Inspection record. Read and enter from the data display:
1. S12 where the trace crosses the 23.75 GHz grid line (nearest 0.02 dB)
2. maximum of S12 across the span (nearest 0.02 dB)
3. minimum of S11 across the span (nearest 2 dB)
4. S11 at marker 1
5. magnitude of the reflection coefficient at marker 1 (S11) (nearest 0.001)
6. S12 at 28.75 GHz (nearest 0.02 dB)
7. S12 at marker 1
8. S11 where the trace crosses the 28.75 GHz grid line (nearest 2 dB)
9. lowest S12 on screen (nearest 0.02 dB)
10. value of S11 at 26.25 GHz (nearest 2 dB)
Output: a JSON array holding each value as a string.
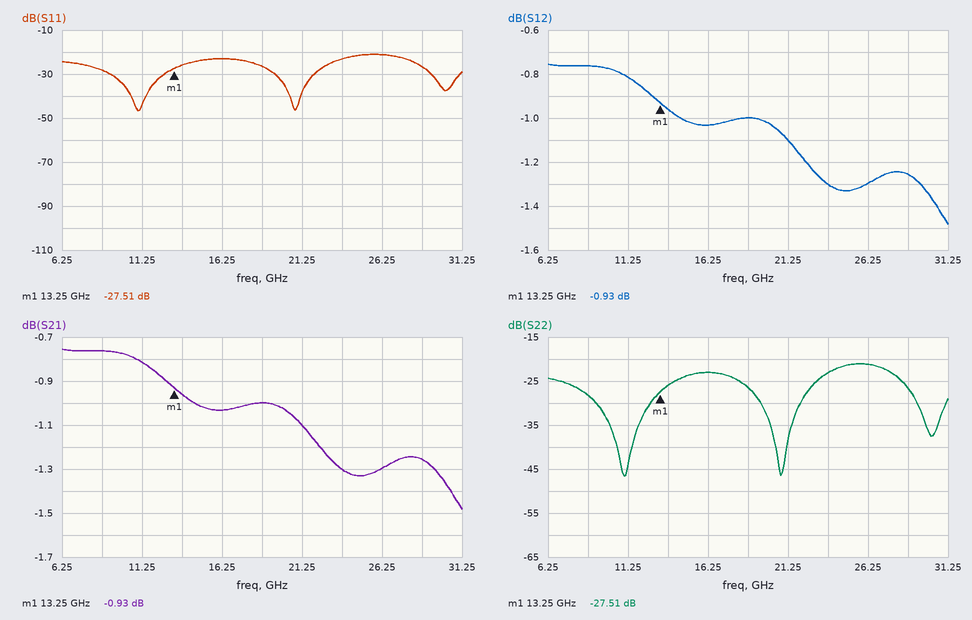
["-1.30 dB", "-0.76 dB", "-46 dB", "-27.51 dB", "0.042", "-1.26 dB", "-0.93 dB", "-26 dB", "-1.48 dB", "-22 dB"]
